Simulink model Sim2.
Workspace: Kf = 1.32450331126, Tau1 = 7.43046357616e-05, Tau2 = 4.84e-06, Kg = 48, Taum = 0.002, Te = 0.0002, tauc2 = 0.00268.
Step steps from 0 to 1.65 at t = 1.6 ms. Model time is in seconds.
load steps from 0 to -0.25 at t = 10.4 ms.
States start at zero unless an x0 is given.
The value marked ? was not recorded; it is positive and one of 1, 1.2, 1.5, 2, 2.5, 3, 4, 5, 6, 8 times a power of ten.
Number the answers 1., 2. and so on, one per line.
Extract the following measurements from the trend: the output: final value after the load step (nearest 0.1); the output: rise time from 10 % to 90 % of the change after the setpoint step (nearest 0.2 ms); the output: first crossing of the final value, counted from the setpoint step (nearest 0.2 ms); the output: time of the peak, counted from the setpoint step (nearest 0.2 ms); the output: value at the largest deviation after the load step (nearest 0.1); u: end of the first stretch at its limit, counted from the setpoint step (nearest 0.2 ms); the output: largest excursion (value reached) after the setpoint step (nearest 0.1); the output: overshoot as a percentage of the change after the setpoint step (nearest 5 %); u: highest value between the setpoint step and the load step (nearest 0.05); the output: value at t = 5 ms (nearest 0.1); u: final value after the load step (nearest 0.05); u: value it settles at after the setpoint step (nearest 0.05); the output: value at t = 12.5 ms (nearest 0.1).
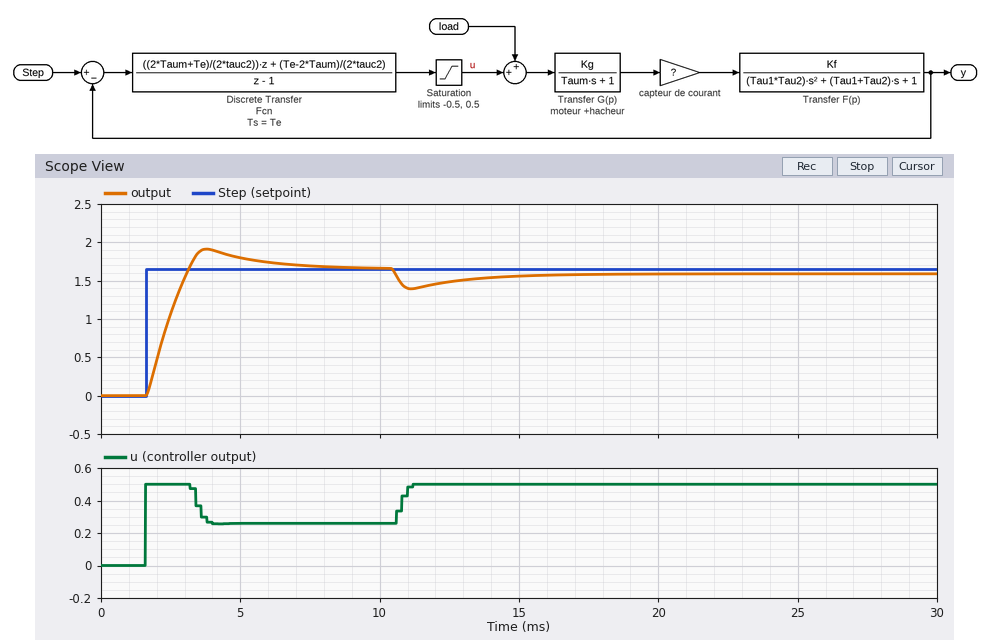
1. 1.6
2. 1.2 ms
3. 1.6 ms
4. 2.2 ms
5. 1.4
6. 1.6 ms
7. 1.9
8. 15 %
9. 0.50
10. 1.8
11. 0.50
12. 0.25
13. 1.5
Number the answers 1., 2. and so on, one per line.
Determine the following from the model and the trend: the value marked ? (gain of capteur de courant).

1. 0.1
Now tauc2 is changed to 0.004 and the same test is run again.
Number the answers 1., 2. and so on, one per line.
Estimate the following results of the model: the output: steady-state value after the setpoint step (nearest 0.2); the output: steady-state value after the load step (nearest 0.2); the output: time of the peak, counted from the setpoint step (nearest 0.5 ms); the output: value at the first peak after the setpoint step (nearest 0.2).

1. 1.6
2. 1.6
3. 2.5 ms
4. 1.8
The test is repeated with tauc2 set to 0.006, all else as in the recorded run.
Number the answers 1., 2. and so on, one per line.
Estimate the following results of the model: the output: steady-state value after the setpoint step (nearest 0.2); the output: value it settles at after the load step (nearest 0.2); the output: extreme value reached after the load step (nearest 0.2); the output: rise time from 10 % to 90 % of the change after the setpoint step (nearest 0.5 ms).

1. 1.6
2. 1.6
3. 1.2
4. 1.5 ms
